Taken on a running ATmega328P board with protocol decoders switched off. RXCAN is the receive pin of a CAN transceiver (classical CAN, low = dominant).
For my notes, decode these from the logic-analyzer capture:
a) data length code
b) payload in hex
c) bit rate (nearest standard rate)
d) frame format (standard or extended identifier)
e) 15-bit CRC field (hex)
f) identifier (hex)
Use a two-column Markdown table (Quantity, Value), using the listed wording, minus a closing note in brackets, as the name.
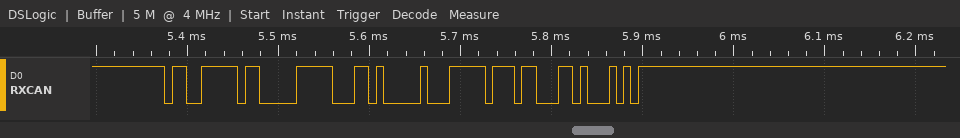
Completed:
| Quantity | Value |
|---|---|
| data length code | 3 |
| payload in hex | CD 00 FF |
| bit rate | 125 kbit/s |
| frame format | standard |
| 15-bit CRC field | 0x31A2 |
| identifier | 0x67F |
